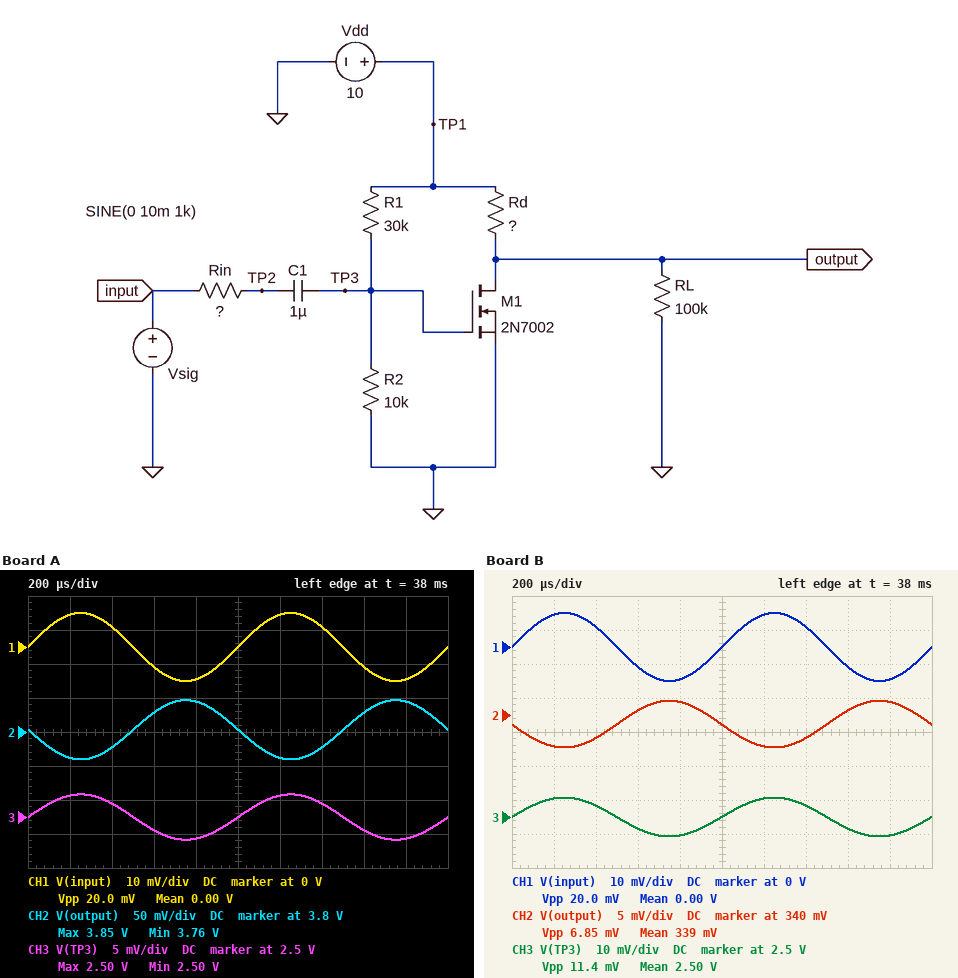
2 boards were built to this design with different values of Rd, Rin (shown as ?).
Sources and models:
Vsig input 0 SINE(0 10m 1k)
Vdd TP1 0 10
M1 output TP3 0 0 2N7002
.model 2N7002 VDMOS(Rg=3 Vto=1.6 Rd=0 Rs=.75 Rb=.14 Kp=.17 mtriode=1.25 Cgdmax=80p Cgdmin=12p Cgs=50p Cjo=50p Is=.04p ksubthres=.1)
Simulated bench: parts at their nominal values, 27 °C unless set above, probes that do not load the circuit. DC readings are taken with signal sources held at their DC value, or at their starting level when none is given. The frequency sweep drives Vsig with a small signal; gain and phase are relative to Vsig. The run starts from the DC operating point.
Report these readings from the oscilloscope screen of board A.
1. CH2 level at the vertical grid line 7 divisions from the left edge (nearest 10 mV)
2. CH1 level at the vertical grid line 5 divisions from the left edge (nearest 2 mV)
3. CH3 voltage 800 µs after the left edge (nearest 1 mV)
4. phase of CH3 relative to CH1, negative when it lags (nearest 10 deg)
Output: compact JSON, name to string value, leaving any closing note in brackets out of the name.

{"CH2 level at the vertical grid line 7 divisions from the left edge": "3.78 V", "CH1 level at the vertical grid line 5 divisions from the left edge": "0 V", "CH3 voltage 800 µs after the left edge": "2.497 V", "phase of CH3 relative to CH1, negative when it lags": "0 deg"}
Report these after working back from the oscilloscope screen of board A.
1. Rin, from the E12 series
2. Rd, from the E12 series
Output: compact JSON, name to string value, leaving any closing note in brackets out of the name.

{"Rin, from the E12 series": "15 kΩ", "Rd, from the E12 series": "100 Ω"}
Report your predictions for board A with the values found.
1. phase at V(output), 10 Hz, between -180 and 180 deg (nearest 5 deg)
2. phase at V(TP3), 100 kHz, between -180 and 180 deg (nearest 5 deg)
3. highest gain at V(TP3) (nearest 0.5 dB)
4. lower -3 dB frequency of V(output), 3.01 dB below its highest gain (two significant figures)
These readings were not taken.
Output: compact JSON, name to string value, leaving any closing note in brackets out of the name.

{"phase at V(output), 10 Hz, between -180 and 180 deg": "-145 deg", "phase at V(TP3), 100 kHz, between -180 and 180 deg": "-55 deg", "highest gain at V(TP3)": "-9.5 dB", "lower -3 dB frequency of V(output), 3.01 dB below its highest gain": "7.1 Hz"}
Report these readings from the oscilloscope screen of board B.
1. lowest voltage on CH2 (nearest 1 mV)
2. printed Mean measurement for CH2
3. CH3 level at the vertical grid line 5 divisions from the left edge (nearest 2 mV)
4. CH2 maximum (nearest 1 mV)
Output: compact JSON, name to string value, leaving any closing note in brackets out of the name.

{"lowest voltage on CH2": "335 mV", "printed Mean measurement for CH2": "339 mV", "CH3 level at the vertical grid line 5 divisions from the left edge": "2.500 V", "CH2 maximum": "342 mV"}
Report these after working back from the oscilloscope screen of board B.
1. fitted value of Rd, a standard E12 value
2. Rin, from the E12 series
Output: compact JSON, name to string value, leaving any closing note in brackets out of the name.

{"fitted value of Rd, a standard E12 value": "220 Ω", "Rin, from the E12 series": "5.6 kΩ"}
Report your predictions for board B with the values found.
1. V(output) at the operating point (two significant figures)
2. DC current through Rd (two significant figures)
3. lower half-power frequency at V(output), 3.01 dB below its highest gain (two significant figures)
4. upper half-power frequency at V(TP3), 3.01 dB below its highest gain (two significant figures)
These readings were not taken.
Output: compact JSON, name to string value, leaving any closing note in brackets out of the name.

{"V(output) at the operating point": "340 mV", "DC current through Rd": "44 mA", "lower half-power frequency at V(output), 3.01 dB below its highest gain": "12 Hz", "upper half-power frequency at V(TP3), 3.01 dB below its highest gain": "280 kHz"}
